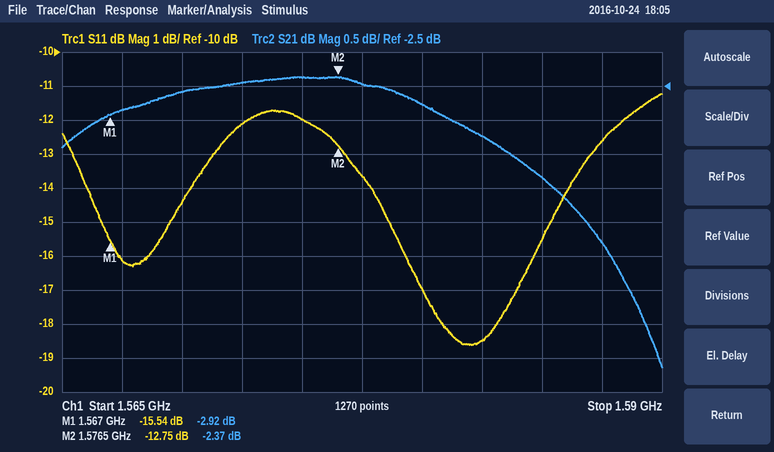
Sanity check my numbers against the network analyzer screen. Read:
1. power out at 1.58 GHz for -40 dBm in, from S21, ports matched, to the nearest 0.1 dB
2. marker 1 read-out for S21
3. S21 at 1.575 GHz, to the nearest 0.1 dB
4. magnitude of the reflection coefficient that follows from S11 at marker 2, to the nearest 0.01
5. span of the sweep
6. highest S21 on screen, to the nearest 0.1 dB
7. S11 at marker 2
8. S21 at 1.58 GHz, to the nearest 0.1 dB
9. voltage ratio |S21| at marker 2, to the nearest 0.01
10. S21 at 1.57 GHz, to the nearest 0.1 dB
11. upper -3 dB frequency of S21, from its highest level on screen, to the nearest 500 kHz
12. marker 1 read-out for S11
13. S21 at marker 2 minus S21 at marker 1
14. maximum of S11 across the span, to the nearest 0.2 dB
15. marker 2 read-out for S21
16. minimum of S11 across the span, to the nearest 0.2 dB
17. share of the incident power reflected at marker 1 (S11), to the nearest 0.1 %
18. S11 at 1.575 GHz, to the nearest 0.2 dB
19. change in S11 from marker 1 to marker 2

-42.8 dBm
-2.92 dB
-2.4 dB
0.23
25 MHz
-2.4 dB
-12.75 dB
-2.8 dB
0.76
-2.6 dB
1.5885 GHz
-15.54 dB
0.55 dB
-11.2 dB
-2.37 dB
-18.6 dB
2.8 %
-12.0 dB
2.79 dB
